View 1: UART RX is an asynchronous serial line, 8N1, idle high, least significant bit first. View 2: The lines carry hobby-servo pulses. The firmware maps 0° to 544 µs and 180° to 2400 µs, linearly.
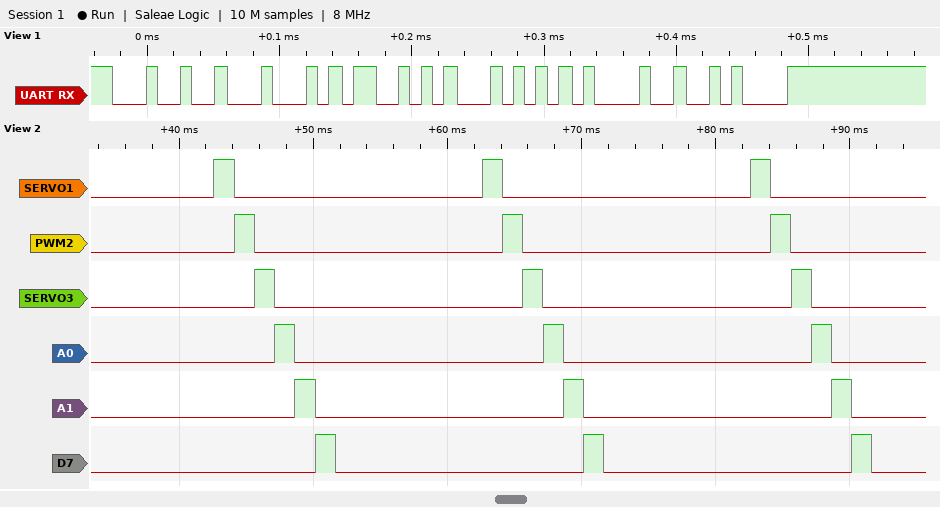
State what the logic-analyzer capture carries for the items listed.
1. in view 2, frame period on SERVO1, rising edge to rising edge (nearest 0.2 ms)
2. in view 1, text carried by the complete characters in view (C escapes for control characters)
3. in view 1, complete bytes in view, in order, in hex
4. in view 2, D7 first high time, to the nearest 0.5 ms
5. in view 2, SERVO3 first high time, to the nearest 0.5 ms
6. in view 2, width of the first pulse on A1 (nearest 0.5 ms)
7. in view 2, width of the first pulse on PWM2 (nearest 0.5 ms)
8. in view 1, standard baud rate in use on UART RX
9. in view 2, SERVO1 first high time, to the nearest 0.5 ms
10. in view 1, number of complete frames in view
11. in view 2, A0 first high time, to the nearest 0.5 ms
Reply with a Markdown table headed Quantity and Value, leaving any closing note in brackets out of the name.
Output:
| Quantity | Value |
|---|---|
| in view 2, frame period on SERVO1, rising edge to rising edge | 20.0 ms |
| in view 1, text carried by the complete characters in view | "$DST!\n" |
| in view 1, complete bytes in view, in order, in hex | 24 44 53 54 21 0A |
| in view 2, D7 first high time, to the nearest 0.5 ms | 1.5 ms |
| in view 2, SERVO3 first high time, to the nearest 0.5 ms | 1.5 ms |
| in view 2, width of the first pulse on A1 | 1.5 ms |
| in view 2, width of the first pulse on PWM2 | 1.5 ms |
| in view 1, standard baud rate in use on UART RX | 115200 baud |
| in view 2, SERVO1 first high time, to the nearest 0.5 ms | 1.5 ms |
| in view 1, number of complete frames in view | 6 |
| in view 2, A0 first high time, to the nearest 0.5 ms | 1.5 ms |
